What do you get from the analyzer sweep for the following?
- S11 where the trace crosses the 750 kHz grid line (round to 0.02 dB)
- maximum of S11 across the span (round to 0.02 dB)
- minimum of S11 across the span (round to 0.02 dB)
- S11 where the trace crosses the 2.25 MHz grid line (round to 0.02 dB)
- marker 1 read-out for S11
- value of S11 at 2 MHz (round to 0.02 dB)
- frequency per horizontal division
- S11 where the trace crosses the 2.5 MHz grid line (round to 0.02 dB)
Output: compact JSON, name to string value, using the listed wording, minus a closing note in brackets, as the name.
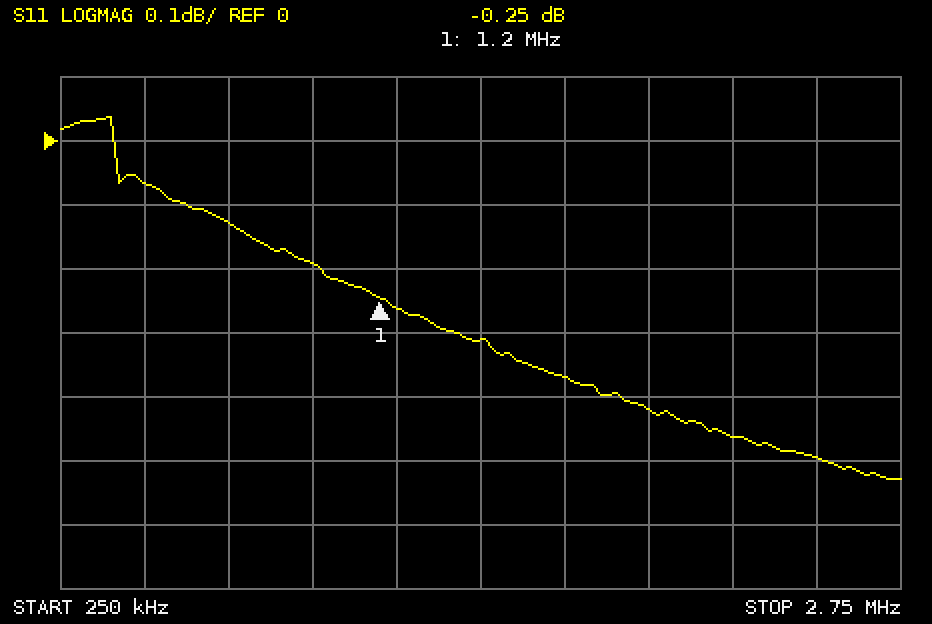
{"S11 where the trace crosses the 750 kHz grid line": "-0.12 dB", "maximum of S11 across the span": "0.04 dB", "minimum of S11 across the span": "-0.52 dB", "S11 where the trace crosses the 2.25 MHz grid line": "-0.46 dB", "marker 1 read-out for S11": "-0.25 dB", "value of S11 at 2 MHz": "-0.42 dB", "frequency per horizontal division": "250 kHz", "S11 where the trace crosses the 2.5 MHz grid line": "-0.50 dB"}
